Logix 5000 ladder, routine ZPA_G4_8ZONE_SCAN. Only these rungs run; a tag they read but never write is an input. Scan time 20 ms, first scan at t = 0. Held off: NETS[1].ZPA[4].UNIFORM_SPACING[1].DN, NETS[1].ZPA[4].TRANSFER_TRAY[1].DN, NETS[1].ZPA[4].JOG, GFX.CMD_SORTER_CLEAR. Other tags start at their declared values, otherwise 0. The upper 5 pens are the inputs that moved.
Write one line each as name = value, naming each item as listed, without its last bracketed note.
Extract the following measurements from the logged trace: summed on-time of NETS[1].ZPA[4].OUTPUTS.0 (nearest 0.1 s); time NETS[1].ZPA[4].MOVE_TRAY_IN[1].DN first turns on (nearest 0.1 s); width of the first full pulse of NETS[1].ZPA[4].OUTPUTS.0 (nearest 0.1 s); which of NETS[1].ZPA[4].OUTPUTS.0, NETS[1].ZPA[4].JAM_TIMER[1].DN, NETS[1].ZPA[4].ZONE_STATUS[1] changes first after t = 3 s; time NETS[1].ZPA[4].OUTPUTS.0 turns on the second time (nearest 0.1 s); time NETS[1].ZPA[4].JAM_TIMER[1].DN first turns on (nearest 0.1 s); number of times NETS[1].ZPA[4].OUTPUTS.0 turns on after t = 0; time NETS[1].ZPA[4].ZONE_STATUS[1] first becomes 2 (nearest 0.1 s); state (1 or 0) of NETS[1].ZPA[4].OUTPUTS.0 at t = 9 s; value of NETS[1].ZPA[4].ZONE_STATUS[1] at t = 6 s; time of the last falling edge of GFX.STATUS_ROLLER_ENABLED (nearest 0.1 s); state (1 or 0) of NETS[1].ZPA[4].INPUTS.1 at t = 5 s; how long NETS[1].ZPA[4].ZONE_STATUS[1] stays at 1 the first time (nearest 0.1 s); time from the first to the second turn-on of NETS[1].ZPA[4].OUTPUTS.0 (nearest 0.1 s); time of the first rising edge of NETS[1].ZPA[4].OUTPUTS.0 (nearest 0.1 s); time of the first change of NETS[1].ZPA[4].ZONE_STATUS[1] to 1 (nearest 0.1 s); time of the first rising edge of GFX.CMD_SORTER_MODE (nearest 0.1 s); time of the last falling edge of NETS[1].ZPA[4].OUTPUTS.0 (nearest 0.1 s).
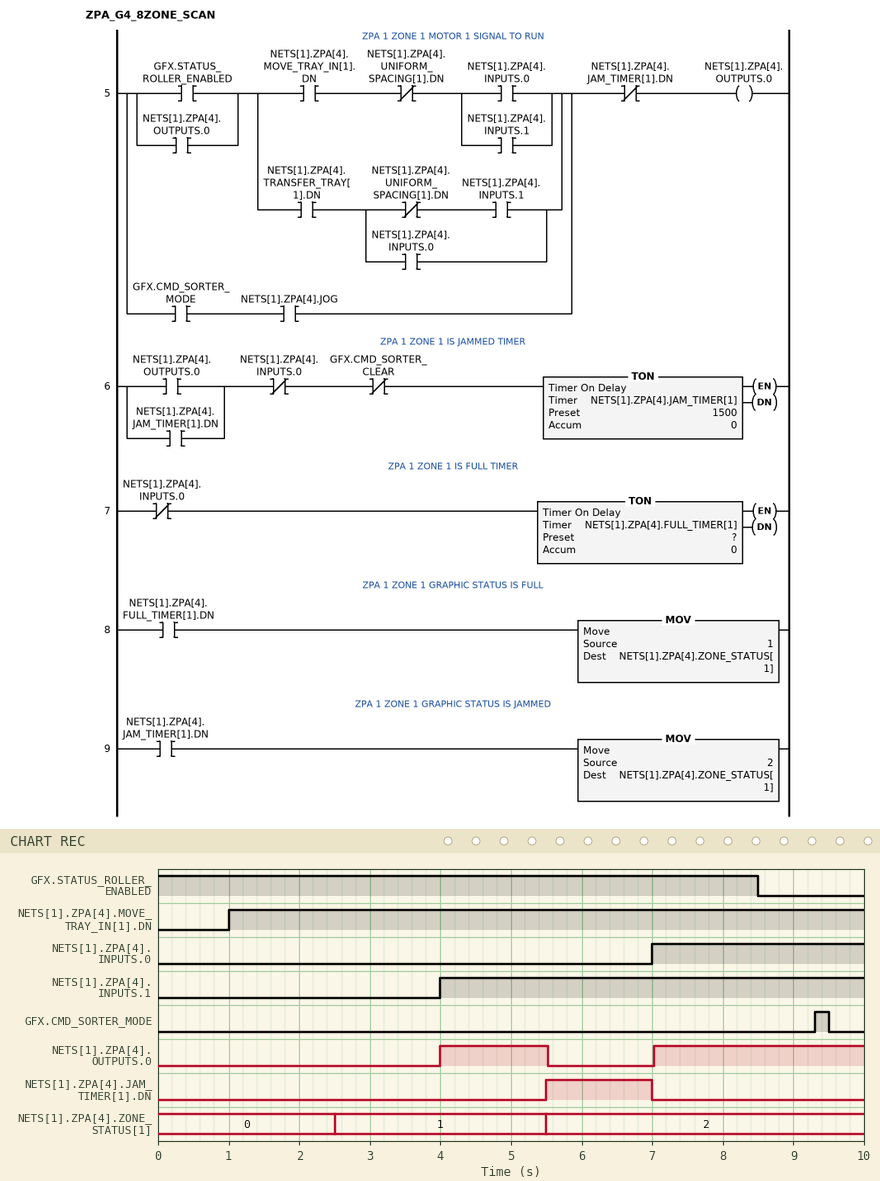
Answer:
summed on-time of NETS[1].ZPA[4].OUTPUTS.0 = 4.5 s
time NETS[1].ZPA[4].MOVE_TRAY_IN[1].DN first turns on = 1.0 s
width of the first full pulse of NETS[1].ZPA[4].OUTPUTS.0 = 1.5 s
which of NETS[1].ZPA[4].OUTPUTS.0, NETS[1].ZPA[4].JAM_TIMER[1].DN, NETS[1].ZPA[4].ZONE_STATUS[1] changes first after t = 3 s = NETS[1].ZPA[4].OUTPUTS.0
time NETS[1].ZPA[4].OUTPUTS.0 turns on the second time = 7.0 s
time NETS[1].ZPA[4].JAM_TIMER[1].DN first turns on = 5.5 s
number of times NETS[1].ZPA[4].OUTPUTS.0 turns on after t = 0 = 2
time NETS[1].ZPA[4].ZONE_STATUS[1] first becomes 2 = 5.5 s
state (1 or 0) of NETS[1].ZPA[4].OUTPUTS.0 at t = 9 s = 1
value of NETS[1].ZPA[4].ZONE_STATUS[1] at t = 6 s = 2
time of the last falling edge of GFX.STATUS_ROLLER_ENABLED = 8.5 s
state (1 or 0) of NETS[1].ZPA[4].INPUTS.1 at t = 5 s = 1
how long NETS[1].ZPA[4].ZONE_STATUS[1] stays at 1 the first time = 3.0 s
time from the first to the second turn-on of NETS[1].ZPA[4].OUTPUTS.0 = 3.0 s
time of the first rising edge of NETS[1].ZPA[4].OUTPUTS.0 = 4.0 s
time of the first change of NETS[1].ZPA[4].ZONE_STATUS[1] to 1 = 2.5 s
time of the first rising edge of GFX.CMD_SORTER_MODE = 9.3 s
time of the last falling edge of NETS[1].ZPA[4].OUTPUTS.0 = 5.5 s
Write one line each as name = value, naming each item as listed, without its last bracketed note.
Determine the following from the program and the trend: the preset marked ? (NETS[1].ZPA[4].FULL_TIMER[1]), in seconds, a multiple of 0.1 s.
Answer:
the preset marked ? (NETS[1].ZPA[4].FULL_TIMER[1]), in seconds, a multiple of 0.1 s = 2.5 s
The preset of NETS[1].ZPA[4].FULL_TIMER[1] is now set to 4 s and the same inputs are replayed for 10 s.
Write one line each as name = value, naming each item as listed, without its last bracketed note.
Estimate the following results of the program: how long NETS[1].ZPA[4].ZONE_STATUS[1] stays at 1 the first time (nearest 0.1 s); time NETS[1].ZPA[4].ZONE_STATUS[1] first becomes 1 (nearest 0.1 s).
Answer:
how long NETS[1].ZPA[4].ZONE_STATUS[1] stays at 1 the first time = 1.5 s
time NETS[1].ZPA[4].ZONE_STATUS[1] first becomes 1 = 4.0 s
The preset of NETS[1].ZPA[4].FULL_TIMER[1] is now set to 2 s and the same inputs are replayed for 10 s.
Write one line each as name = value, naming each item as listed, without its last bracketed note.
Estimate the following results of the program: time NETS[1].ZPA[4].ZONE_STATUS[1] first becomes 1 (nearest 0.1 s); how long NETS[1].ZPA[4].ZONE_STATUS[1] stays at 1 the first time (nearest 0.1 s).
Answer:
time NETS[1].ZPA[4].ZONE_STATUS[1] first becomes 1 = 2.0 s
how long NETS[1].ZPA[4].ZONE_STATUS[1] stays at 1 the first time = 3.5 s
